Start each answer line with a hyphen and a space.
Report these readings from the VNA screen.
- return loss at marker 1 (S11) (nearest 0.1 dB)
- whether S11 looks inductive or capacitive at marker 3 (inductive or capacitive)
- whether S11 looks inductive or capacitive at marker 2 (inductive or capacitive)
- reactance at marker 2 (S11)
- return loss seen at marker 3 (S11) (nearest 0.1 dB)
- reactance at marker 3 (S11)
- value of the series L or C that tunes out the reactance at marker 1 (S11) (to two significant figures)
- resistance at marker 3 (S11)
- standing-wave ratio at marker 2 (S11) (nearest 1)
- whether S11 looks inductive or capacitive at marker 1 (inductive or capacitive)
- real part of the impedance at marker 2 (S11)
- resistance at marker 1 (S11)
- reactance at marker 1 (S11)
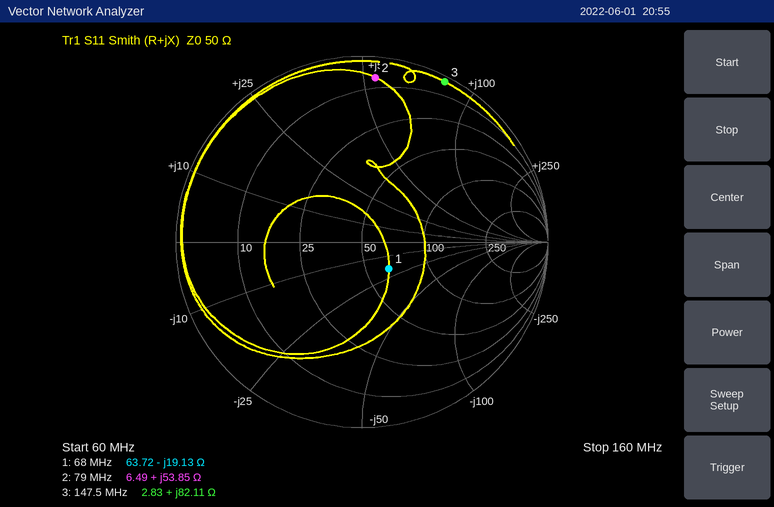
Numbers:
- 13.8 dB
- inductive
- inductive
- +53.85 Ω
- 0.3 dB
- +82.11 Ω
- 45 nH
- 2.83 Ω
- 17
- capacitive
- 6.49 Ω
- 63.72 Ω
- -19.13 Ω
